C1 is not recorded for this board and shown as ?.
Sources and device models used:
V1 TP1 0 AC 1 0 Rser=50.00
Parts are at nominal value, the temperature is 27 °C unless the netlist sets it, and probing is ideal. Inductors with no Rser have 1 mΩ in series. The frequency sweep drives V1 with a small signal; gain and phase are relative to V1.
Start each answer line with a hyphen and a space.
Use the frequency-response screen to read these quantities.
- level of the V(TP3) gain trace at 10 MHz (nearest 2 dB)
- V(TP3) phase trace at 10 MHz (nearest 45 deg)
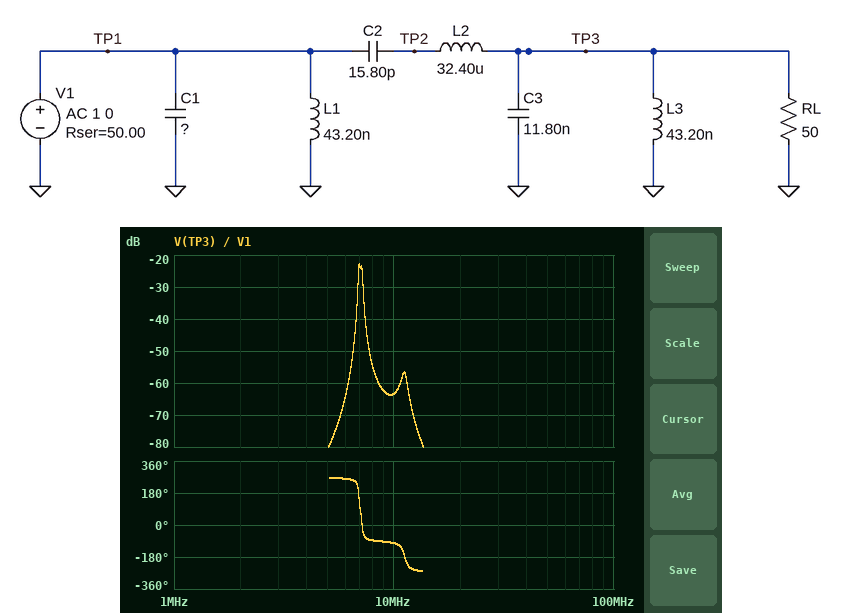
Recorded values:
- -64 dB
- -90 deg
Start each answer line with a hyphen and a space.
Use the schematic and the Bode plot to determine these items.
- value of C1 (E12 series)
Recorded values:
- 4.7 nF
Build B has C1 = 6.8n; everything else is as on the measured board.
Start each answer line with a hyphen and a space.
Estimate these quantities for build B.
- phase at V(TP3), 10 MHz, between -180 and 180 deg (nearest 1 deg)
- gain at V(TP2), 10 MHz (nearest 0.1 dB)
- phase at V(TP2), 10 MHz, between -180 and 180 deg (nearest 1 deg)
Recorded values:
- 112 deg
- -3.8 dB
- -71 deg
